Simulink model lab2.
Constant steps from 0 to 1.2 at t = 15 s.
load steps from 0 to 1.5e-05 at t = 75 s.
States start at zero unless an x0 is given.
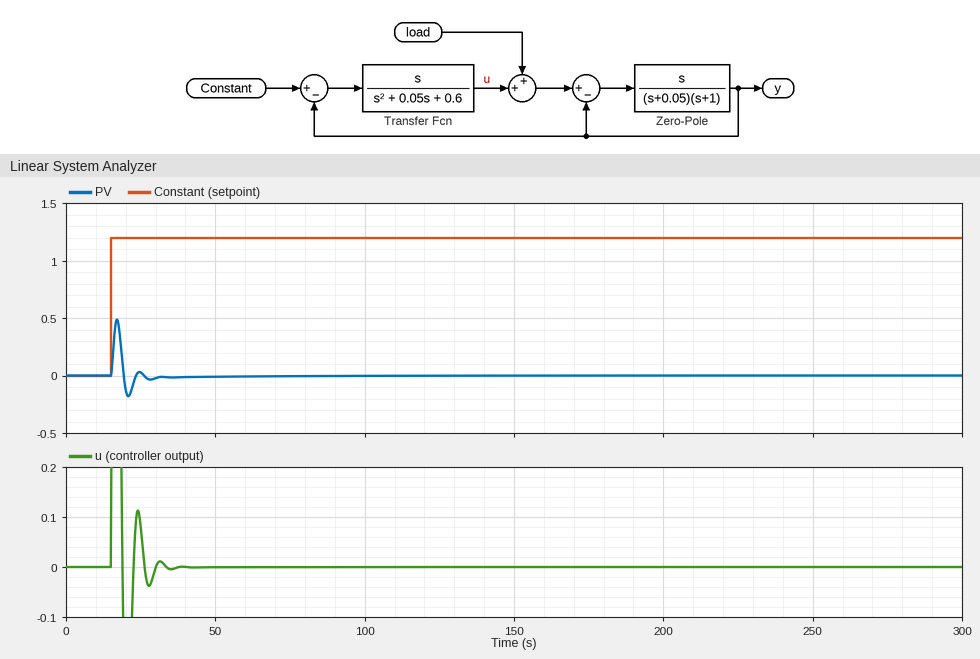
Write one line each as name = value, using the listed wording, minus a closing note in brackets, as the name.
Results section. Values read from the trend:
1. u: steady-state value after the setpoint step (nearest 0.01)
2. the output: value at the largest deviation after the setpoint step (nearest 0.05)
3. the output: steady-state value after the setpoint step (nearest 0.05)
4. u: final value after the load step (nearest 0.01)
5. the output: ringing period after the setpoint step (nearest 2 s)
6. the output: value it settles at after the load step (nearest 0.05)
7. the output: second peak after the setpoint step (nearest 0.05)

u: steady-state value after the setpoint step = 0.00
the output: value at the largest deviation after the setpoint step = 0.50
the output: steady-state value after the setpoint step = 0.00
u: final value after the load step = 0.00
the output: ringing period after the setpoint step = 8 s
the output: value it settles at after the load step = 0.00
the output: second peak after the setpoint step = 0.05
